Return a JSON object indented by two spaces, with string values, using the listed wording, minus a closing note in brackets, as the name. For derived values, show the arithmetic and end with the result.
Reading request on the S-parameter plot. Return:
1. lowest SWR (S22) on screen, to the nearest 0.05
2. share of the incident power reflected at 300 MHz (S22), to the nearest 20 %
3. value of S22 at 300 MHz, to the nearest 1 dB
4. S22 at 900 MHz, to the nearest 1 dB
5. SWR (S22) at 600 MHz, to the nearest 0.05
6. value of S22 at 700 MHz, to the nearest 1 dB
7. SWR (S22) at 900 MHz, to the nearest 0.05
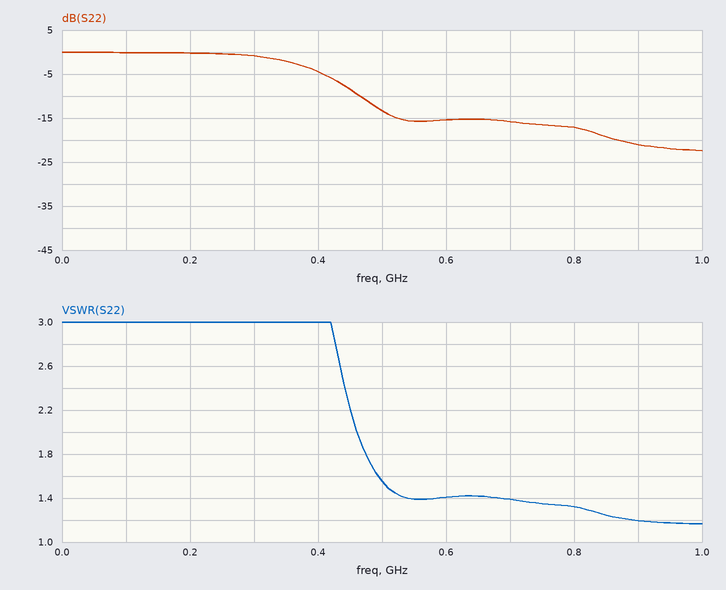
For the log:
{
  "lowest SWR (S22) on screen, to the nearest 0.05": "1.15",
  "share of the incident power reflected at 300 MHz (S22), to the nearest 20 %": "10^(-1/10) ≈ 79.4 %, so 80 % to the nearest 20 %",
  "value of S22 at 300 MHz, to the nearest 1 dB": "-1 dB",
  "S22 at 900 MHz, to the nearest 1 dB": "-21 dB",
  "SWR (S22) at 600 MHz, to the nearest 0.05": "1.40",
  "value of S22 at 700 MHz, to the nearest 1 dB": "-16 dB",
  "SWR (S22) at 900 MHz, to the nearest 0.05": "1.20"
}
